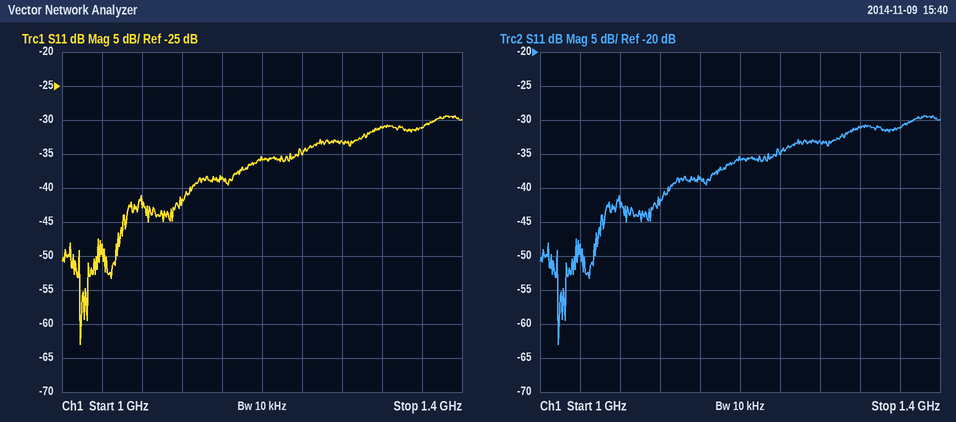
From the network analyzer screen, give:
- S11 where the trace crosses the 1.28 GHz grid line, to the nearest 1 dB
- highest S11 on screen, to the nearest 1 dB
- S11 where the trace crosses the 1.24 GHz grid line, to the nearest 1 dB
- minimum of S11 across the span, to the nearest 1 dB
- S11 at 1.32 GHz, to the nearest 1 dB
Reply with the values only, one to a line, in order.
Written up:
-33 dB
-29 dB
-35 dB
-63 dB
-31 dB
